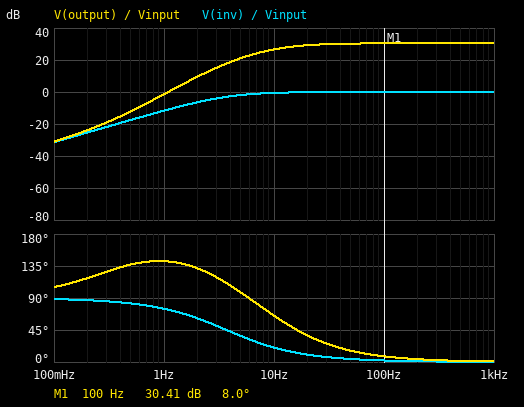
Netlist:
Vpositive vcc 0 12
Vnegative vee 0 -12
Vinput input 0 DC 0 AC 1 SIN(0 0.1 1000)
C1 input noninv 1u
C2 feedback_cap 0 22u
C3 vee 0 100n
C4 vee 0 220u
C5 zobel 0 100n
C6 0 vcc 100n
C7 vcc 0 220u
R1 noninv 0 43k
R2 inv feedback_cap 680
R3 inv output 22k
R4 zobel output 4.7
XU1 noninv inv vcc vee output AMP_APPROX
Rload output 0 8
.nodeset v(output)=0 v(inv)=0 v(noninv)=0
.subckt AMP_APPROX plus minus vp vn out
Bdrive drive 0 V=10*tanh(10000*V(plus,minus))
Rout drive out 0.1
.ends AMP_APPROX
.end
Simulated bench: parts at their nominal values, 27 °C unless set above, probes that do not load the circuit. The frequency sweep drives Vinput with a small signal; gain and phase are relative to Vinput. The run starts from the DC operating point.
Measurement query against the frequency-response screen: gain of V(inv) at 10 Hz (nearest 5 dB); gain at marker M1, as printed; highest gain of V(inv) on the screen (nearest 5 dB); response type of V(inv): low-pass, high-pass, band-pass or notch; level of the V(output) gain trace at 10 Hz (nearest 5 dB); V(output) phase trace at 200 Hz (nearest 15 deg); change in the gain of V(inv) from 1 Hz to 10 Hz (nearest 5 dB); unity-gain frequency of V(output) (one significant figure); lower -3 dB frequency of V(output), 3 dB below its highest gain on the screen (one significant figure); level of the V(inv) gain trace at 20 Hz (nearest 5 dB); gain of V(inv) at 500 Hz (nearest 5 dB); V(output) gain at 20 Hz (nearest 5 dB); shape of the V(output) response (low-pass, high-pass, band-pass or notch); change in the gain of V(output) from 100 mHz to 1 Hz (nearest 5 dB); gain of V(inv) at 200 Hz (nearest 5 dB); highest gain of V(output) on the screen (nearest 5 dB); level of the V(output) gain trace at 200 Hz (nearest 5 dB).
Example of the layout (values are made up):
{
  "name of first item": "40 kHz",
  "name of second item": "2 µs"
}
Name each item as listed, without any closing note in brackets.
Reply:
{
  "gain of V(inv) at 10 Hz": "0 dB",
  "gain at marker M1, as printed": "30.41 dB",
  "highest gain of V(inv) on the screen": "0 dB",
  "response type of V(inv): low-pass, high-pass, band-pass or notch": "high-pass",
  "level of the V(output) gain trace at 10 Hz": "25 dB",
  "V(output) phase trace at 200 Hz": "0 deg",
  "change in the gain of V(inv) from 1 Hz to 10 Hz": "10 dB",
  "unity-gain frequency of V(output)": "1 Hz",
  "lower -3 dB frequency of V(output), 3 dB below its highest gain on the screen": "10 Hz",
  "level of the V(inv) gain trace at 20 Hz": "0 dB",
  "gain of V(inv) at 500 Hz": "0 dB",
  "V(output) gain at 20 Hz": "30 dB",
  "shape of the V(output) response": "high-pass",
  "change in the gain of V(output) from 100 mHz to 1 Hz": "30 dB",
  "gain of V(inv) at 200 Hz": "0 dB",
  "highest gain of V(output) on the screen": "30 dB",
  "level of the V(output) gain trace at 200 Hz": "30 dB"
}
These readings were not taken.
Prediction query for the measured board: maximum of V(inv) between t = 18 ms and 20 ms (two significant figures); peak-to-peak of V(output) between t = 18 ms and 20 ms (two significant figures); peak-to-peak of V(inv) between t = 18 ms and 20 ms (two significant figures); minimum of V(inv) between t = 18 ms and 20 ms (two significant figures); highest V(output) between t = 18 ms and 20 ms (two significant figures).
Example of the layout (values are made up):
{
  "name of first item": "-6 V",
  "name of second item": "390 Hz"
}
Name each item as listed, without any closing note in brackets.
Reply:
{
  "maximum of V(inv) between t = 18 ms and 20 ms": "100 mV",
  "peak-to-peak of V(output) between t = 18 ms and 20 ms": "6.7 V",
  "peak-to-peak of V(inv) between t = 18 ms and 20 ms": "200 mV",
  "minimum of V(inv) between t = 18 ms and 20 ms": "-100 mV",
  "highest V(output) between t = 18 ms and 20 ms": "3.3 V"
}
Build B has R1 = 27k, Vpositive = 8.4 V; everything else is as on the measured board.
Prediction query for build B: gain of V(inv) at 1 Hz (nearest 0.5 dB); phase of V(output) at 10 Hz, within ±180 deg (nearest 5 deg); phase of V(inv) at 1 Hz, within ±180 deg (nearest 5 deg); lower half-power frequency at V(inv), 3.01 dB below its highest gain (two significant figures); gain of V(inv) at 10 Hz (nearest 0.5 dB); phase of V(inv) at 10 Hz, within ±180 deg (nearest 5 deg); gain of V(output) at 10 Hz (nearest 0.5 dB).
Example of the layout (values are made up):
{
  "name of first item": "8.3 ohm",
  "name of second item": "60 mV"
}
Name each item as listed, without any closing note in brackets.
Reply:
{
  "gain of V(inv) at 1 Hz": "-15.5 dB",
  "phase of V(output) at 10 Hz, within ±180 deg": "75 deg",
  "phase of V(inv) at 1 Hz, within ±180 deg": "80 deg",
  "lower half-power frequency at V(inv), 3.01 dB below its highest gain": "5.9 Hz",
  "gain of V(inv) at 10 Hz": "-1.5 dB",
  "phase of V(inv) at 10 Hz, within ±180 deg": "30 deg",
  "gain of V(output) at 10 Hz": "26.0 dB"
}
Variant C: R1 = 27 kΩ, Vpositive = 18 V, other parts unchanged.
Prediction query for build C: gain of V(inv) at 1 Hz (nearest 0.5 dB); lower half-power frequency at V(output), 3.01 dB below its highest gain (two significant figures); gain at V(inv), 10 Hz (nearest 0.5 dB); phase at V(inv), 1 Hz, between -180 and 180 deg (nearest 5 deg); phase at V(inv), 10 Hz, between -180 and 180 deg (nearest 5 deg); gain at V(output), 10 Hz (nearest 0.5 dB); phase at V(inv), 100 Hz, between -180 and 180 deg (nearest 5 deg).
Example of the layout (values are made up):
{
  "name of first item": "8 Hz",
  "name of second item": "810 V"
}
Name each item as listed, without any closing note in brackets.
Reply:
{
  "gain of V(inv) at 1 Hz": "-15.5 dB",
  "lower half-power frequency at V(output), 3.01 dB below its highest gain": "13 Hz",
  "gain at V(inv), 10 Hz": "-1.5 dB",
  "phase at V(inv), 1 Hz, between -180 and 180 deg": "80 deg",
  "phase at V(inv), 10 Hz, between -180 and 180 deg": "30 deg",
  "gain at V(output), 10 Hz": "26.0 dB",
  "phase at V(inv), 100 Hz, between -180 and 180 deg": "5 deg"
}
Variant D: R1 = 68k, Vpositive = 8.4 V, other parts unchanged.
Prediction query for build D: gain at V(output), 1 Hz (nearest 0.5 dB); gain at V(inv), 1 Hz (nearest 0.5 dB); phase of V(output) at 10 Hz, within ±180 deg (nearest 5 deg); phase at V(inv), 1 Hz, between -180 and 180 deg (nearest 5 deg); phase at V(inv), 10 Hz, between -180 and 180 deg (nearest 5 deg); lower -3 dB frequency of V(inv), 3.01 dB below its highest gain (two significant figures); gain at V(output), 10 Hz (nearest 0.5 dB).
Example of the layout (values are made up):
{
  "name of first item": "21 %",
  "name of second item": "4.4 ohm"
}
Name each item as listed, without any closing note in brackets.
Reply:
{
  "gain at V(output), 1 Hz": "2.0 dB",
  "gain at V(inv), 1 Hz": "-8.0 dB",
  "phase of V(output) at 10 Hz, within ±180 deg": "60 deg",
  "phase at V(inv), 1 Hz, between -180 and 180 deg": "65 deg",
  "phase at V(inv), 10 Hz, between -180 and 180 deg": "15 deg",
  "lower -3 dB frequency of V(inv), 3.01 dB below its highest gain": "2.3 Hz",
  "gain at V(output), 10 Hz": "27.0 dB"
}
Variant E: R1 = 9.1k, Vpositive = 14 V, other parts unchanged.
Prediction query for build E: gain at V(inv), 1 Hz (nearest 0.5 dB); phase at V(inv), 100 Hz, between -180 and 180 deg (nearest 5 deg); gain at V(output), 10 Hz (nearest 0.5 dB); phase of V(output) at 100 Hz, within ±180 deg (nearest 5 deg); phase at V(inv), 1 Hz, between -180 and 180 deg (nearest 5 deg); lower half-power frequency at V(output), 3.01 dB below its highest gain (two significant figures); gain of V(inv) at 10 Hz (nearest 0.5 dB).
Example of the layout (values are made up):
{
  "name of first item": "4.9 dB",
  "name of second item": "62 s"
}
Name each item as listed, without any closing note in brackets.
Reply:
{
  "gain at V(inv), 1 Hz": "-25.0 dB",
  "phase at V(inv), 100 Hz, between -180 and 180 deg": "10 deg",
  "gain at V(output), 10 Hz": "21.0 dB",
  "phase of V(output) at 100 Hz, within ±180 deg": "15 deg",
  "phase at V(inv), 1 Hz, between -180 and 180 deg": "85 deg",
  "lower half-power frequency at V(output), 3.01 dB below its highest gain": "22 Hz",
  "gain of V(inv) at 10 Hz": "-6.0 dB"
}
